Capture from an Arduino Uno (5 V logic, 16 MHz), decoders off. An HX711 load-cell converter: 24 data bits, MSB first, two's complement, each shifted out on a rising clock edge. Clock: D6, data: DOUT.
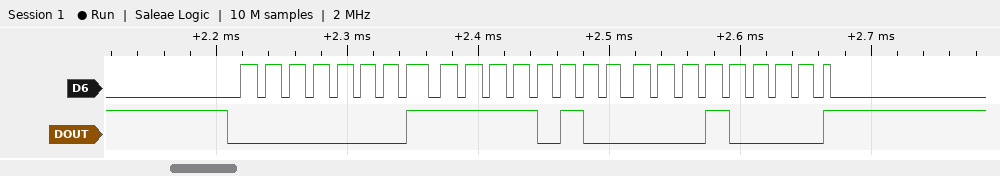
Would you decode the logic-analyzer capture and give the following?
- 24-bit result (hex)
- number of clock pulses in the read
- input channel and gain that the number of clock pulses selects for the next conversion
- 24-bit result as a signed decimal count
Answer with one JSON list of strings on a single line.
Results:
["0x01F410", "25", "channel A, gain 128", "128016"]
